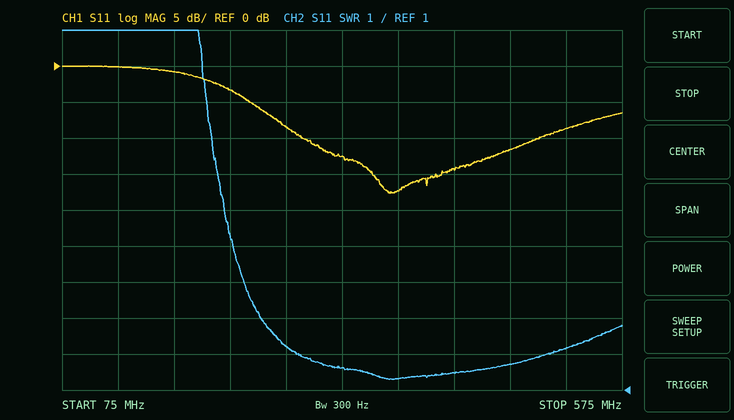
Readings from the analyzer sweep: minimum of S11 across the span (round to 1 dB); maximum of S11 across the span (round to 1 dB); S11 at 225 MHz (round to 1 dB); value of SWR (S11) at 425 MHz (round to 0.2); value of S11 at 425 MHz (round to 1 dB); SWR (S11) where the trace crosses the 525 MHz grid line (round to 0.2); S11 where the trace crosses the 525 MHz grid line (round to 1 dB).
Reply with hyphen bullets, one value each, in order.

- -18 dB
- 0 dB
- -3 dB
- 1.4
- -14 dB
- 2.2
- -9 dB
